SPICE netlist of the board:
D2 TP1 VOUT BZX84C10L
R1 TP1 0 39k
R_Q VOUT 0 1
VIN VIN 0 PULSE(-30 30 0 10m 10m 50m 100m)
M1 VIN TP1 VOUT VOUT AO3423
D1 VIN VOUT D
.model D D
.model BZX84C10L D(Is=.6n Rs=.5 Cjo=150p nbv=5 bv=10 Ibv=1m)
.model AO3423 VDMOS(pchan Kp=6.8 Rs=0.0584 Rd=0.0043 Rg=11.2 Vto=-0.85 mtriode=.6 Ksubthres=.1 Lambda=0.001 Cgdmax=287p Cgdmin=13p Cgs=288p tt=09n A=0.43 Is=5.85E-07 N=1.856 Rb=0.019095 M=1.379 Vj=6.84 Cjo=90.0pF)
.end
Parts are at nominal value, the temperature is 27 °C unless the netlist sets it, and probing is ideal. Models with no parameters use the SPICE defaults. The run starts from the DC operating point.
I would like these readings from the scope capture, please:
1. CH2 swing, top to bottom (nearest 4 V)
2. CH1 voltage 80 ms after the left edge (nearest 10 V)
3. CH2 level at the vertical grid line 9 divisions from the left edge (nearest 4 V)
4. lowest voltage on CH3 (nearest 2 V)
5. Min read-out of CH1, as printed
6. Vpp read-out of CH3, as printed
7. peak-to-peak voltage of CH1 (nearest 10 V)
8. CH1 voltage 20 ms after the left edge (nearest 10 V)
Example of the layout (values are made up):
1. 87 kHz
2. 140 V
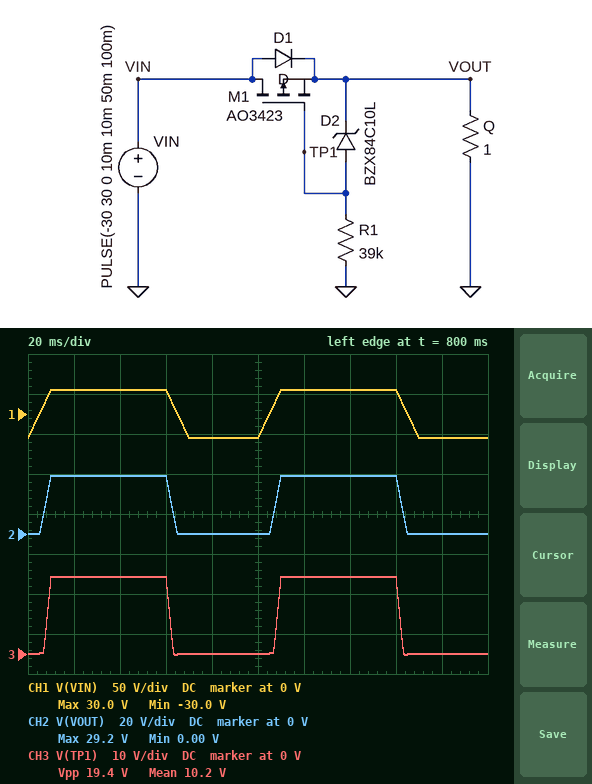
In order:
1. 28 V
2. -30 V
3. 0 V
4. 0 V
5. -30.0 V
6. 19.4 V
7. 60 V
8. 30 V
